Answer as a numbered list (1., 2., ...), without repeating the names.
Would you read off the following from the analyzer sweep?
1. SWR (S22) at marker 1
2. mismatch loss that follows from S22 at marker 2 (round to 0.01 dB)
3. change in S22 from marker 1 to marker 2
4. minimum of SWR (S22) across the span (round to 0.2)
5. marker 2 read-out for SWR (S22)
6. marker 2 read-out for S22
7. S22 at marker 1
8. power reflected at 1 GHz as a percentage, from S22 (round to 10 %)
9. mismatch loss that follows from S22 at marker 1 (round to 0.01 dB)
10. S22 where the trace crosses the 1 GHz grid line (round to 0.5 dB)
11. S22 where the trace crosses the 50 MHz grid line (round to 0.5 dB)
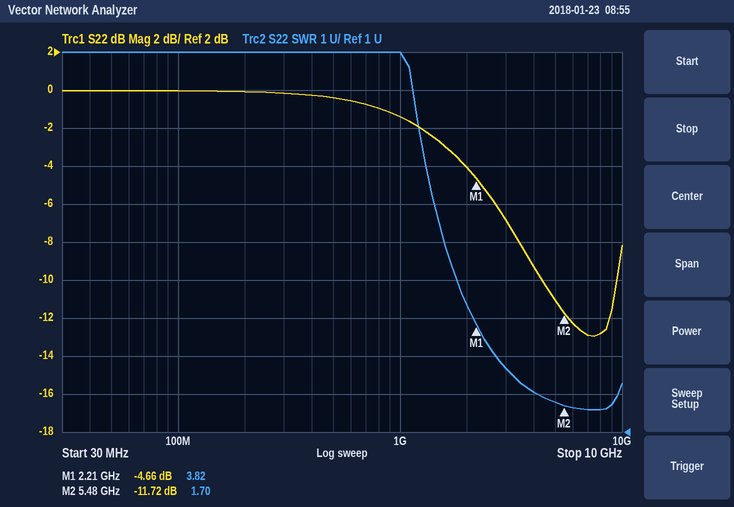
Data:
1. 3.82
2. 0.30 dB
3. -7.06 dB
4. 1.6
5. 1.70
6. -11.72 dB
7. -4.66 dB
8. 70 %
9. 1.82 dB
10. -1.5 dB
11. 0.0 dB
